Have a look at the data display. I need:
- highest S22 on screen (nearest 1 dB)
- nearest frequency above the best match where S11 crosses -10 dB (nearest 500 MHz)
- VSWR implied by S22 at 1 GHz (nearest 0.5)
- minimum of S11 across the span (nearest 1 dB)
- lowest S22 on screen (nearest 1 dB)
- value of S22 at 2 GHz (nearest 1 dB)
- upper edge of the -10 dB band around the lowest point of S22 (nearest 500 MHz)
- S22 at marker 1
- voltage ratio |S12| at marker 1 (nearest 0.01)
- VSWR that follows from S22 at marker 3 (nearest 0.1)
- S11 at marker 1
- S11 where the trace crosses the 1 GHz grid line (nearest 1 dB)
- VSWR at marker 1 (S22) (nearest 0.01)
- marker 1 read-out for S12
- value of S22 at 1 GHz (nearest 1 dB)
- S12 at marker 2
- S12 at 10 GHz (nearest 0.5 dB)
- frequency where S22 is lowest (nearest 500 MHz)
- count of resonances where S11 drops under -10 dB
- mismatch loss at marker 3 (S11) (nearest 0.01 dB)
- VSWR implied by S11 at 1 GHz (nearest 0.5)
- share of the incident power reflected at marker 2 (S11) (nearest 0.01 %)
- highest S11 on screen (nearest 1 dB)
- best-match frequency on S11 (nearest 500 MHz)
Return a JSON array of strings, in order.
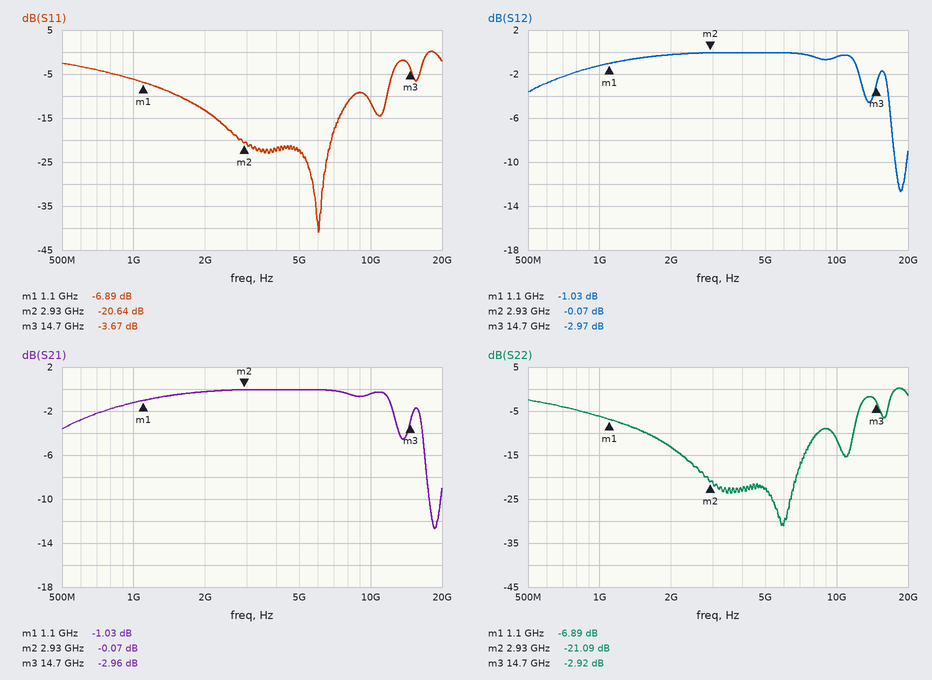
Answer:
["0 dB", "8.5 GHz", "3.0", "-41 dB", "-31 dB", "-13 dB", "8.5 GHz", "-6.89 dB", "0.89", "6.0", "-6.89 dB", "-6 dB", "2.65", "-1.03 dB", "-6 dB", "-0.07 dB", "-0.5 dB", "6.0 GHz", "2", "2.44 dB", "3.0", "0.86 %", "0 dB", "6.0 GHz"]
